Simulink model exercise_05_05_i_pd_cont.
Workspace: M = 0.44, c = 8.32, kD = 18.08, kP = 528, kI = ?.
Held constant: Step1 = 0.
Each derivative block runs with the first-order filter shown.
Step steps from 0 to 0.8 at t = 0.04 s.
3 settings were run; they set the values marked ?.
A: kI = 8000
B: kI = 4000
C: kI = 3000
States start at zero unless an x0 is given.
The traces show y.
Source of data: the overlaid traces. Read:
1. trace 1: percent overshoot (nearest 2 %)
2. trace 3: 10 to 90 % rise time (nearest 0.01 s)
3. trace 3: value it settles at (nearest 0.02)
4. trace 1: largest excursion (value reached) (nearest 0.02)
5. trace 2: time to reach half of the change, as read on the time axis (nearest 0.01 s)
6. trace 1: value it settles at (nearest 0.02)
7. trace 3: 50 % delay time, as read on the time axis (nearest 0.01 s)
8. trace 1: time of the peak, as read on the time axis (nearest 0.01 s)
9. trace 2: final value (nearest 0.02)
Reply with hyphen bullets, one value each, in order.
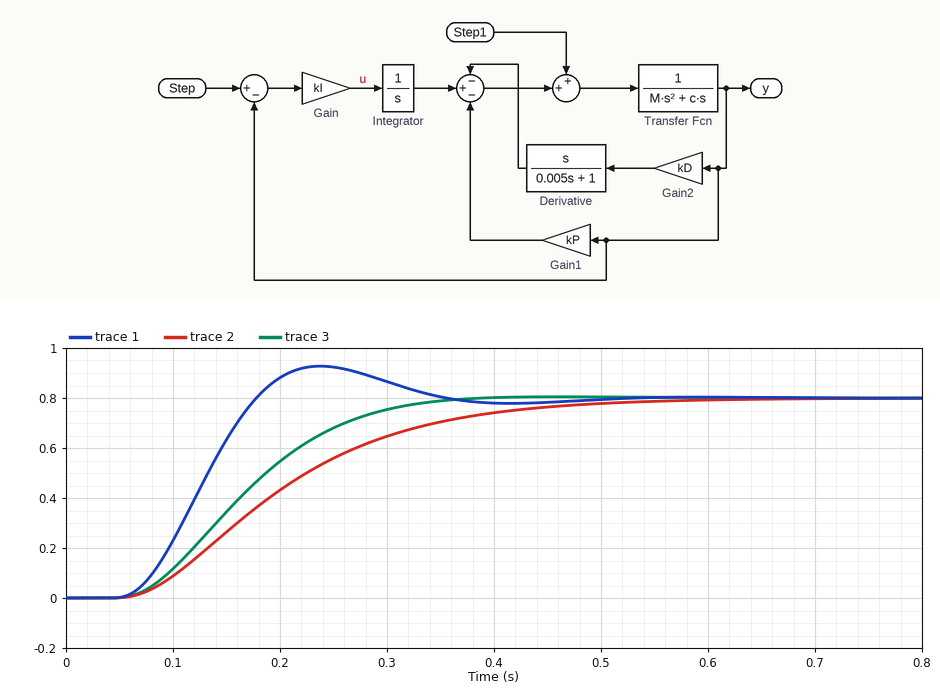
- 16 %
- 0.18 s
- 0.80
- 0.92
- 0.19 s
- 0.80
- 0.16 s
- 0.24 s
- 0.80
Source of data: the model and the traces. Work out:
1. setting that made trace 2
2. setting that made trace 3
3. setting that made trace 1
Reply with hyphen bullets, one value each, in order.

- C
- B
- A
